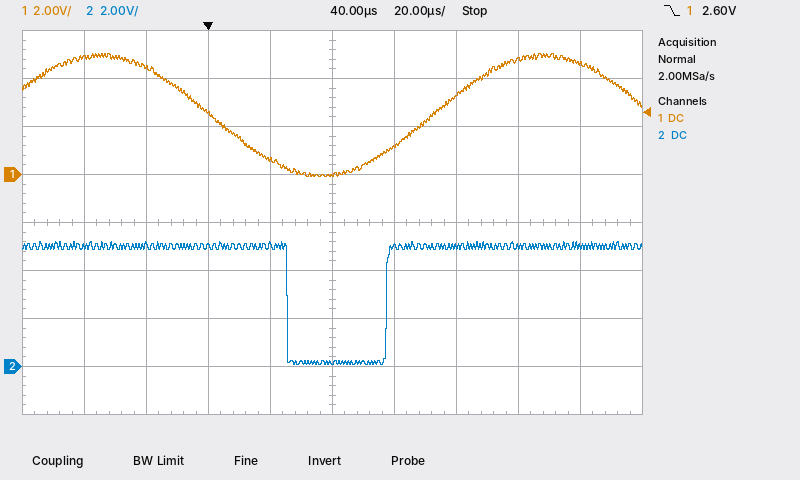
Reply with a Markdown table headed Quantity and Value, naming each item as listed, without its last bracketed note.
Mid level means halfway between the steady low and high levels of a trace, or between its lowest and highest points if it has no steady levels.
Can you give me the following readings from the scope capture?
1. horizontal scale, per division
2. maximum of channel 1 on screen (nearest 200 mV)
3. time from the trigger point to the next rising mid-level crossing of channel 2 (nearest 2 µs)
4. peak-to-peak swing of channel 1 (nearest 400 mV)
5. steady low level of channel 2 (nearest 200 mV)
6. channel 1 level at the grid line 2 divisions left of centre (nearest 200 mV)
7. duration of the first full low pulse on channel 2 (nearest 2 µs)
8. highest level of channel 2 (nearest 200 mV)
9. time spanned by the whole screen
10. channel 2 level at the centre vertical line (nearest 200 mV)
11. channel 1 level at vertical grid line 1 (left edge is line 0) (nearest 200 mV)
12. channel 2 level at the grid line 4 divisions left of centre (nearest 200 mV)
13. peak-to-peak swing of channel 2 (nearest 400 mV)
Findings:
| Quantity | Value |
|---|---|
| horizontal scale, per division | 20 µs |
| maximum of channel 1 on screen | 5.0 V |
| time from the trigger point to the next rising mid-level crossing of channel 2 | 58 µs |
| peak-to-peak swing of channel 1 | 5.2 V |
| steady low level of channel 2 | 200 mV |
| channel 1 level at the grid line 2 divisions left of centre | 2.6 V |
| duration of the first full low pulse on channel 2 | 32 µs |
| highest level of channel 2 | 5.2 V |
| time spanned by the whole screen | 200 µs |
| channel 2 level at the centre vertical line | 200 mV |
| channel 1 level at vertical grid line 1 (left edge is line 0) | 4.8 V |
| channel 2 level at the grid line 4 divisions left of centre | 5.0 V |
| peak-to-peak swing of channel 2 | 5.2 V |
